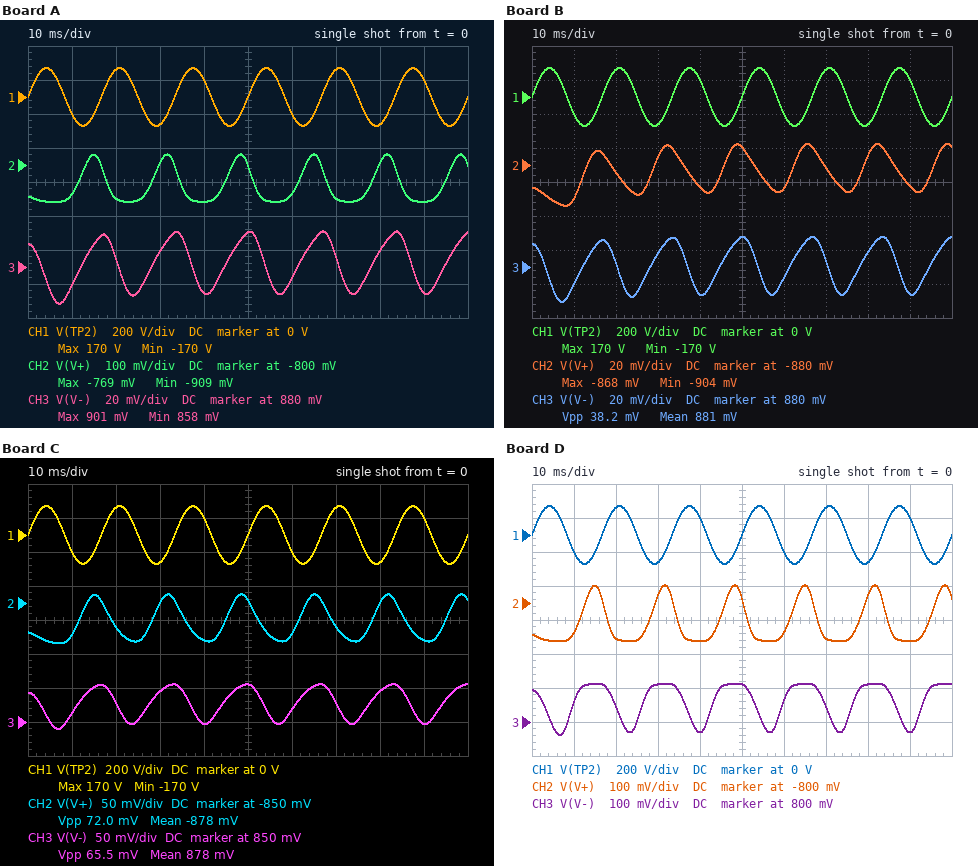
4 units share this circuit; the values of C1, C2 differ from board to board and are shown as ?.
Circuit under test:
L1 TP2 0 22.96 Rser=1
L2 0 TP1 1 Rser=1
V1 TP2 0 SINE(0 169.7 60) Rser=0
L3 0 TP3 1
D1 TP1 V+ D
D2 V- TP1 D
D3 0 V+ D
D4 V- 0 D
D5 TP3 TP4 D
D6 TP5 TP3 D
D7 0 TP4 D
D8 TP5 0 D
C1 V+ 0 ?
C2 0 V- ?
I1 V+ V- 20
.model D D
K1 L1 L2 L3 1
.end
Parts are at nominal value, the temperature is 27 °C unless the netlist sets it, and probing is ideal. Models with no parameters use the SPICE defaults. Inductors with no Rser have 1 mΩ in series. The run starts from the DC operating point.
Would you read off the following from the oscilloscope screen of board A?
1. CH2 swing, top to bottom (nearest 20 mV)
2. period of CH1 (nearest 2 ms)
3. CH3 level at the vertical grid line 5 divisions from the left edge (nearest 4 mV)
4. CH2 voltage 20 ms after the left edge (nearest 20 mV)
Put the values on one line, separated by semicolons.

140 mV; 16 ms; 900 mV; -900 mV
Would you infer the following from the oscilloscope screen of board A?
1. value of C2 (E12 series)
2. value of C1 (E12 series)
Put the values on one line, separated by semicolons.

2.7 F; 470 mF
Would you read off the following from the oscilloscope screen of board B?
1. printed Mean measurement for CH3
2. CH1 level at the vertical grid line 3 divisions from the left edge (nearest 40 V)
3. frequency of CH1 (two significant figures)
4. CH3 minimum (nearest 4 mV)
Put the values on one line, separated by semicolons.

881 mV; -160 V; 60 Hz; 860 mV
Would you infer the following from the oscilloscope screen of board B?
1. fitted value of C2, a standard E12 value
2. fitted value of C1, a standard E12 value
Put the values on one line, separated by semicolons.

2.7 F; 3.3 F
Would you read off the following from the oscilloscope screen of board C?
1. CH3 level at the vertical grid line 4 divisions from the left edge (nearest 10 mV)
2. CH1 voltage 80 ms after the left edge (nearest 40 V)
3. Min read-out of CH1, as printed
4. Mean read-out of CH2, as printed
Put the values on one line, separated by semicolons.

850 mV; -160 V; -170 V; -878 mV
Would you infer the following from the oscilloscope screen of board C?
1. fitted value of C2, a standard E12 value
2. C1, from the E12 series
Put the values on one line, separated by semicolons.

1.5 F; 1.2 F
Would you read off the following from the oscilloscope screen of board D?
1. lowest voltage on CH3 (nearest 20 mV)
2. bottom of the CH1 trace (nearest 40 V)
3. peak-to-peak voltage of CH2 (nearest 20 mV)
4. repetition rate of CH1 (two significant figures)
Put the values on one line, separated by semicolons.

760 mV; -160 V; 160 mV; 60 Hz
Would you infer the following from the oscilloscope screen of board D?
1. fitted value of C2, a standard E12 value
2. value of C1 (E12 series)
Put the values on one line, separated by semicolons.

470 mF; 390 mF
